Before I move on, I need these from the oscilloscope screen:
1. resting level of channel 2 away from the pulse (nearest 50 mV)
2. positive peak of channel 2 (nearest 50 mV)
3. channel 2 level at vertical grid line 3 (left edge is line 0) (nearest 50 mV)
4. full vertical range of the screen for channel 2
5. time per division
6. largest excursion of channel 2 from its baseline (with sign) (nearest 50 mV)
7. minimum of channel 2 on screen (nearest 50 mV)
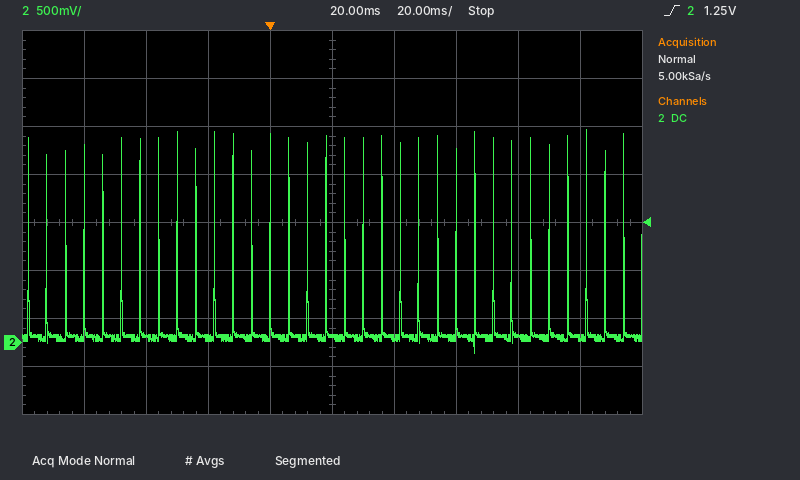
50 mV
2.20 V
50 mV
4 V
20 ms
+2.15 V
-100 mV
